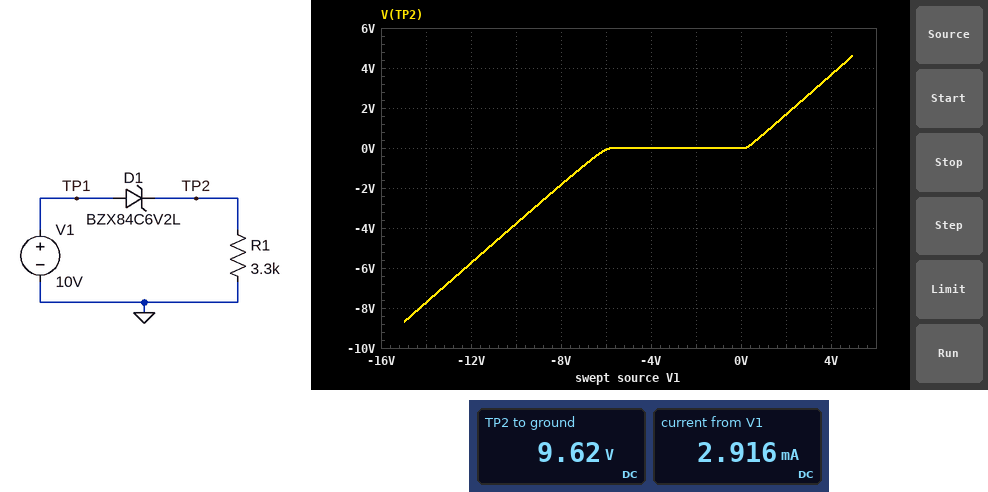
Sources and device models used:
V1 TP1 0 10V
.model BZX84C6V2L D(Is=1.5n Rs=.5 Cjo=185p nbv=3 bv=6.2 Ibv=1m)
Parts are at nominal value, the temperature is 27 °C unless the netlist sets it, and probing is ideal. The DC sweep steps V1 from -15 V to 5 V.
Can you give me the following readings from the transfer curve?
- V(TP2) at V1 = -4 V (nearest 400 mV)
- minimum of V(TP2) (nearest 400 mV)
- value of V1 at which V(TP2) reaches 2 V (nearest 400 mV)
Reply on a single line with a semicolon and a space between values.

0 V; -8.8 V; 2.4 V
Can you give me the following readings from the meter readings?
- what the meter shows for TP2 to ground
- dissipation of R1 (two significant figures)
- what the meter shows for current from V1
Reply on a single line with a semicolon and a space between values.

9.62 V; 28 mW; 2.916 mA
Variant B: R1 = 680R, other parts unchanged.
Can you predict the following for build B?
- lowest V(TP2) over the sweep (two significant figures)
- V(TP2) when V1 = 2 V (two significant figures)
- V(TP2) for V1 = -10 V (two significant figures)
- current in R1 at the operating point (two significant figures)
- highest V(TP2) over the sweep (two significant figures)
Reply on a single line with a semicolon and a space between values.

-8.6 V; 1.6 V; -3.7 V; 14 mA; 4.6 V
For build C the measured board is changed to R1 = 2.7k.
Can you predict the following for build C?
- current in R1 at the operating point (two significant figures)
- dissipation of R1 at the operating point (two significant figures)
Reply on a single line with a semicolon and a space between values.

3.6 mA; 34 mW
